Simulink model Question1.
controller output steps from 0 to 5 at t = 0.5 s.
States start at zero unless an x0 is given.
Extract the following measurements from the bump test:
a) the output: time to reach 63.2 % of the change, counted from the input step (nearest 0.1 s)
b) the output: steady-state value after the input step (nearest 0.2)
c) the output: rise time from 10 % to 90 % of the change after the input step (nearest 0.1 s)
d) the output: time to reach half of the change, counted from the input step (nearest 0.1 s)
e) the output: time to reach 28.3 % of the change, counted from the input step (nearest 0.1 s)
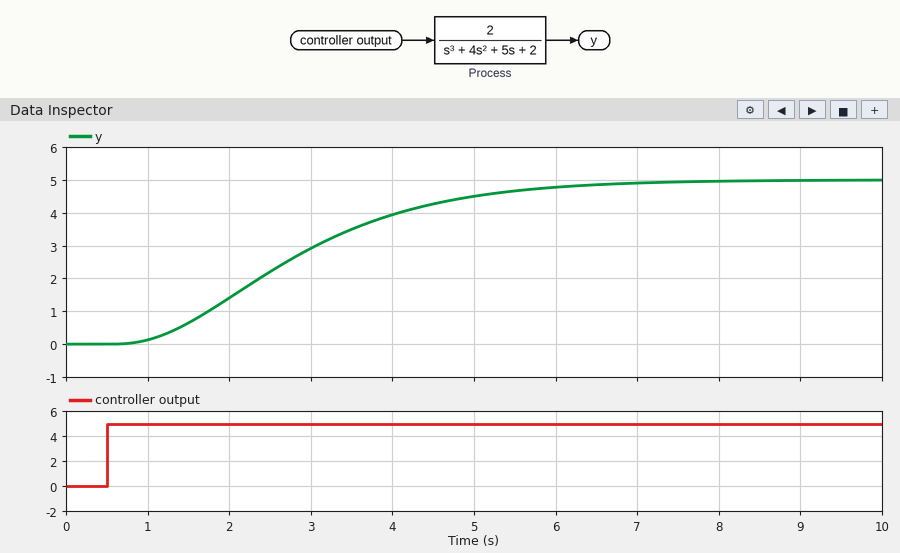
2.7 s
5.0
3.6 s
2.2 s
1.5 s
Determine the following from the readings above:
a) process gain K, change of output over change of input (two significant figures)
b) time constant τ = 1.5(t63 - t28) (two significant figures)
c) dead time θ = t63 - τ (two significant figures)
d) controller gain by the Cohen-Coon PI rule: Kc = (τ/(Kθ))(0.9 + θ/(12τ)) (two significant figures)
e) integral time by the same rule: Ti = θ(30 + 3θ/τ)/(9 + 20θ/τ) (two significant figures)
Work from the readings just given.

1.0
1.8 s
0.90 s
1.9
1.5 s
